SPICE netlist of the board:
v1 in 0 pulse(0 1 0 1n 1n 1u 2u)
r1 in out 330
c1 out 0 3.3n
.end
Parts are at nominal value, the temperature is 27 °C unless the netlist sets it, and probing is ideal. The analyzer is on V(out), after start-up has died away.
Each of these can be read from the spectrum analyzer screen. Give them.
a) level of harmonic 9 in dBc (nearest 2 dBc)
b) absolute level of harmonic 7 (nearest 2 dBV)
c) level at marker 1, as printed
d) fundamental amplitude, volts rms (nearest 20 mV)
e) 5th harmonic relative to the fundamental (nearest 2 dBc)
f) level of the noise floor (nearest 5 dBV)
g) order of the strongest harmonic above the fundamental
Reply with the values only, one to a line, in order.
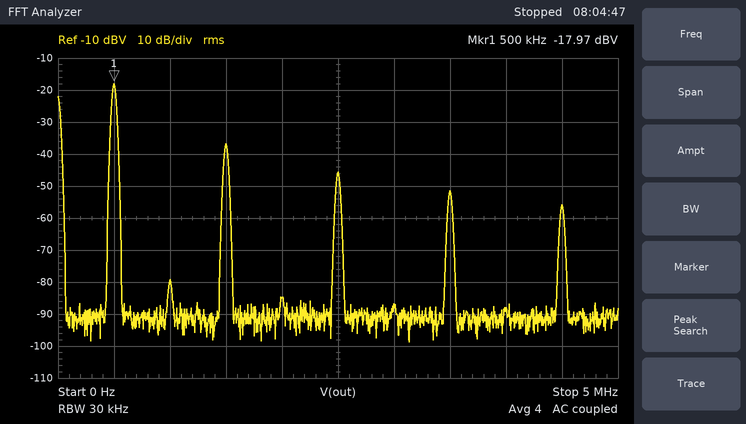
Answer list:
-38 dBc
-52 dBV
-17.97 dBV
120 mV
-28 dBc
-90 dBV
3
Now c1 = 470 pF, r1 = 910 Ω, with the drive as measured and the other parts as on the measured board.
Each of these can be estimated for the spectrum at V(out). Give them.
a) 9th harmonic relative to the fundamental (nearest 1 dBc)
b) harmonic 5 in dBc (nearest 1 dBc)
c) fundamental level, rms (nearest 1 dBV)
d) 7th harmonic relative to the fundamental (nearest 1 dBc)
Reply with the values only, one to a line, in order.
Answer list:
-36 dBc
-26 dBc
-11 dBV
-32 dBc
